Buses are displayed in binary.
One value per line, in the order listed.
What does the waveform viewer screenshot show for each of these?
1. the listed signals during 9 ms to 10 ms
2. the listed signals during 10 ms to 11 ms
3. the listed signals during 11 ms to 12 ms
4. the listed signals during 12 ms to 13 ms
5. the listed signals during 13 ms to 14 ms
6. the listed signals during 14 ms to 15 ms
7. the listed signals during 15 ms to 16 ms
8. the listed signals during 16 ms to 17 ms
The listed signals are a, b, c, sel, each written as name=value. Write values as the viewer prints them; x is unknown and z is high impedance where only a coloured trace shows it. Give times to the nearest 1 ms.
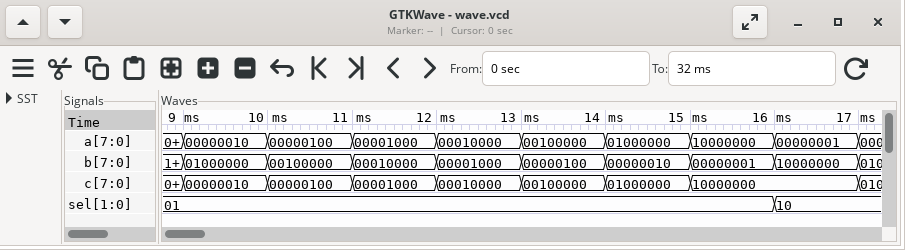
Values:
a=00000010, b=01000000, c=00000010, sel=01
a=00000100, b=00100000, c=00000100, sel=01
a=00001000, b=00010000, c=00001000, sel=01
a=00010000, b=00001000, c=00010000, sel=01
a=00100000, b=00000100, c=00100000, sel=01
a=01000000, b=00000010, c=01000000, sel=01
a=10000000, b=00000001, c=10000000, sel=01
a=00000001, b=10000000, c=10000000, sel=10
